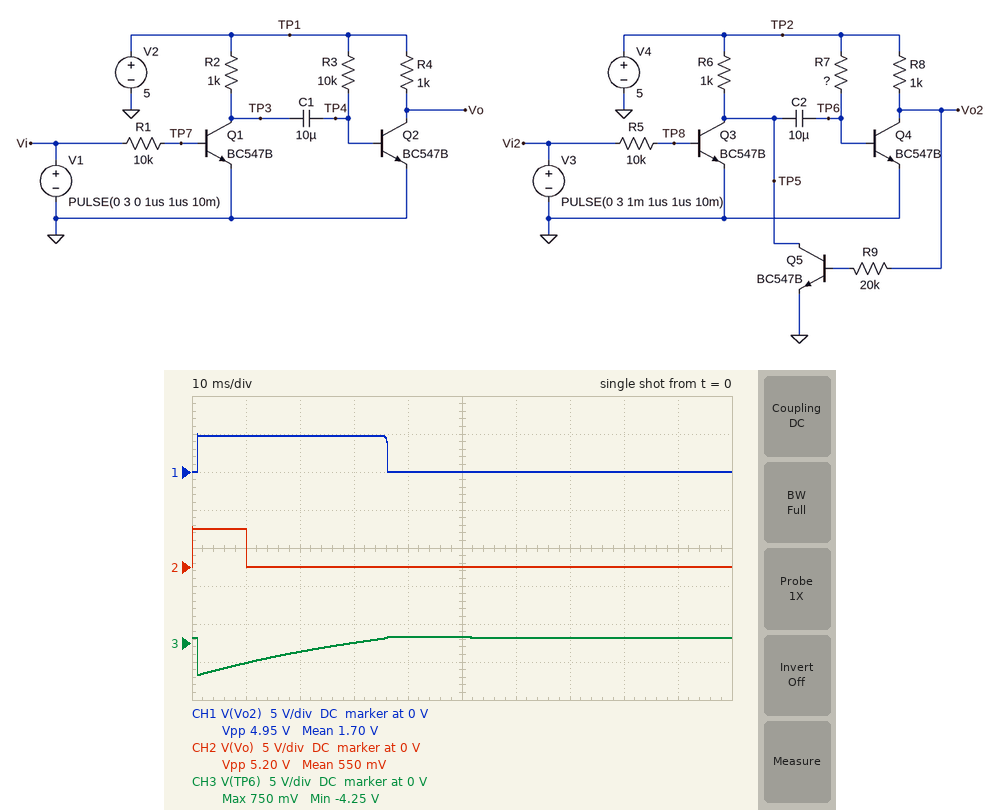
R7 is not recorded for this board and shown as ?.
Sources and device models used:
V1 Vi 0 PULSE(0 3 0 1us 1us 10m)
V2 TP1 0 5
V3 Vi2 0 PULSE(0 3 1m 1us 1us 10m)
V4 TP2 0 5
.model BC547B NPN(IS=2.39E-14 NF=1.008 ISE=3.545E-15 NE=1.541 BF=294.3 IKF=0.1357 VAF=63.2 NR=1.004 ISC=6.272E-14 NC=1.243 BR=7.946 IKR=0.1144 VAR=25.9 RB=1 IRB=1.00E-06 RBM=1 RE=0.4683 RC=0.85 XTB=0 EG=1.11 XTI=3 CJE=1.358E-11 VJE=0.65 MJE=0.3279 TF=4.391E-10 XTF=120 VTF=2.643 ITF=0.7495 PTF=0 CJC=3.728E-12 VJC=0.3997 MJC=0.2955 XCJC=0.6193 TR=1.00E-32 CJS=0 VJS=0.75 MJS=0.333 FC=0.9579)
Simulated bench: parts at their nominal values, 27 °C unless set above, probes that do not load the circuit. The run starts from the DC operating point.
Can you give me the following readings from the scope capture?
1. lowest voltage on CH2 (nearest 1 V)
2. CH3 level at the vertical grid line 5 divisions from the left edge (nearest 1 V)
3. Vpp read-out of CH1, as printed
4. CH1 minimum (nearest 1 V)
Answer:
0 V
1 V
4.95 V
0 V
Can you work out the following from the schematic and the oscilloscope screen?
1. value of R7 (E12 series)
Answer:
4.7 kΩ
